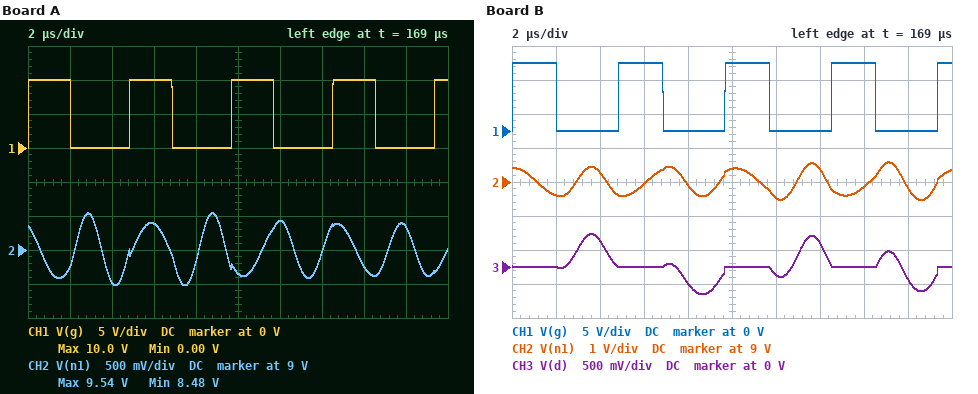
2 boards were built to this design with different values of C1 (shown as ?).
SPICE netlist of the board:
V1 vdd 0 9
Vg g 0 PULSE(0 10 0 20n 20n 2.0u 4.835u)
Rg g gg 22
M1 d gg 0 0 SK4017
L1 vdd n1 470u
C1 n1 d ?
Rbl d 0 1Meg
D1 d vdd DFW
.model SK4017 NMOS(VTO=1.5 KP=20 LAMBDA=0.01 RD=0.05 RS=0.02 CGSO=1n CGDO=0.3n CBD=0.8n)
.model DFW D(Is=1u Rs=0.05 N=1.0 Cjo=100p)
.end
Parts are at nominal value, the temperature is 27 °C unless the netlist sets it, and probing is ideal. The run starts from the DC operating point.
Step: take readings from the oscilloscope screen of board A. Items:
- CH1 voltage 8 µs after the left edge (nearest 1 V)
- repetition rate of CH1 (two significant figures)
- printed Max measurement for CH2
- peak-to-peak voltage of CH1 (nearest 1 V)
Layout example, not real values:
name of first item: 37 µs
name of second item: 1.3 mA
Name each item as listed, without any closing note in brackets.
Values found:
CH1 voltage 8 µs after the left edge: 0 V
repetition rate of CH1: 210 kHz
printed Max measurement for CH2: 9.54 V
peak-to-peak voltage of CH1: 10 V
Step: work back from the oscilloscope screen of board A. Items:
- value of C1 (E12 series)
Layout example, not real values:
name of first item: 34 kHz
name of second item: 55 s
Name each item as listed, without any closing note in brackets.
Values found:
value of C1: 680 pF
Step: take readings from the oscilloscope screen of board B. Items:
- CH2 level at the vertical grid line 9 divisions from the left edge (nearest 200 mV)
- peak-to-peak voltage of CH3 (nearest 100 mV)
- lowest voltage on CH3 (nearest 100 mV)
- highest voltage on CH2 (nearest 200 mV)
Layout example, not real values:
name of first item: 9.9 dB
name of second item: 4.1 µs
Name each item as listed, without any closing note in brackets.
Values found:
CH2 level at the vertical grid line 9 divisions from the left edge: 8.8 V
peak-to-peak voltage of CH3: 900 mV
lowest voltage on CH3: -400 mV
highest voltage on CH2: 9.6 V
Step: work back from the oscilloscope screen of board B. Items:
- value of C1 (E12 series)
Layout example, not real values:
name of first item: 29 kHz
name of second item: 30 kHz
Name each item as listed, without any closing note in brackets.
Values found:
value of C1: 1 nF
